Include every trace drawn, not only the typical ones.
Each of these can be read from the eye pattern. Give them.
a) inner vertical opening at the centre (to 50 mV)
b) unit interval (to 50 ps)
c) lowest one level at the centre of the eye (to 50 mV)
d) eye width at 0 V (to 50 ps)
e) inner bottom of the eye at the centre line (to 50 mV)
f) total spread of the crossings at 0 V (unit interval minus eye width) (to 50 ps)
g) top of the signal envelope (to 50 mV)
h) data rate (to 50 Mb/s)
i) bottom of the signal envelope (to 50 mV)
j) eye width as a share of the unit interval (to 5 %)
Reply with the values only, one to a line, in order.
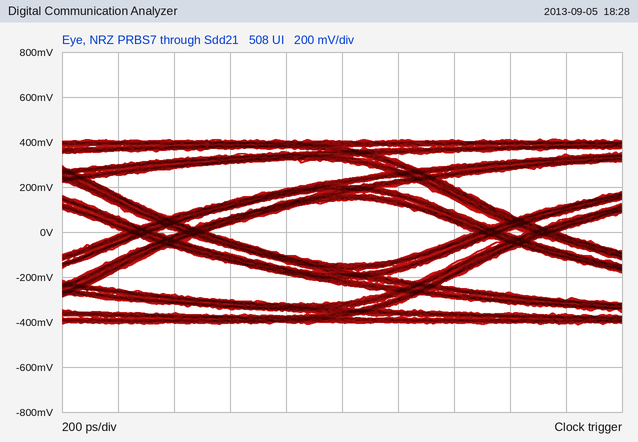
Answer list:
300 mV
1.25 ns
150 mV
950 ps
-150 mV
300 ps
400 mV
800 Mb/s
-400 mV
75 %
